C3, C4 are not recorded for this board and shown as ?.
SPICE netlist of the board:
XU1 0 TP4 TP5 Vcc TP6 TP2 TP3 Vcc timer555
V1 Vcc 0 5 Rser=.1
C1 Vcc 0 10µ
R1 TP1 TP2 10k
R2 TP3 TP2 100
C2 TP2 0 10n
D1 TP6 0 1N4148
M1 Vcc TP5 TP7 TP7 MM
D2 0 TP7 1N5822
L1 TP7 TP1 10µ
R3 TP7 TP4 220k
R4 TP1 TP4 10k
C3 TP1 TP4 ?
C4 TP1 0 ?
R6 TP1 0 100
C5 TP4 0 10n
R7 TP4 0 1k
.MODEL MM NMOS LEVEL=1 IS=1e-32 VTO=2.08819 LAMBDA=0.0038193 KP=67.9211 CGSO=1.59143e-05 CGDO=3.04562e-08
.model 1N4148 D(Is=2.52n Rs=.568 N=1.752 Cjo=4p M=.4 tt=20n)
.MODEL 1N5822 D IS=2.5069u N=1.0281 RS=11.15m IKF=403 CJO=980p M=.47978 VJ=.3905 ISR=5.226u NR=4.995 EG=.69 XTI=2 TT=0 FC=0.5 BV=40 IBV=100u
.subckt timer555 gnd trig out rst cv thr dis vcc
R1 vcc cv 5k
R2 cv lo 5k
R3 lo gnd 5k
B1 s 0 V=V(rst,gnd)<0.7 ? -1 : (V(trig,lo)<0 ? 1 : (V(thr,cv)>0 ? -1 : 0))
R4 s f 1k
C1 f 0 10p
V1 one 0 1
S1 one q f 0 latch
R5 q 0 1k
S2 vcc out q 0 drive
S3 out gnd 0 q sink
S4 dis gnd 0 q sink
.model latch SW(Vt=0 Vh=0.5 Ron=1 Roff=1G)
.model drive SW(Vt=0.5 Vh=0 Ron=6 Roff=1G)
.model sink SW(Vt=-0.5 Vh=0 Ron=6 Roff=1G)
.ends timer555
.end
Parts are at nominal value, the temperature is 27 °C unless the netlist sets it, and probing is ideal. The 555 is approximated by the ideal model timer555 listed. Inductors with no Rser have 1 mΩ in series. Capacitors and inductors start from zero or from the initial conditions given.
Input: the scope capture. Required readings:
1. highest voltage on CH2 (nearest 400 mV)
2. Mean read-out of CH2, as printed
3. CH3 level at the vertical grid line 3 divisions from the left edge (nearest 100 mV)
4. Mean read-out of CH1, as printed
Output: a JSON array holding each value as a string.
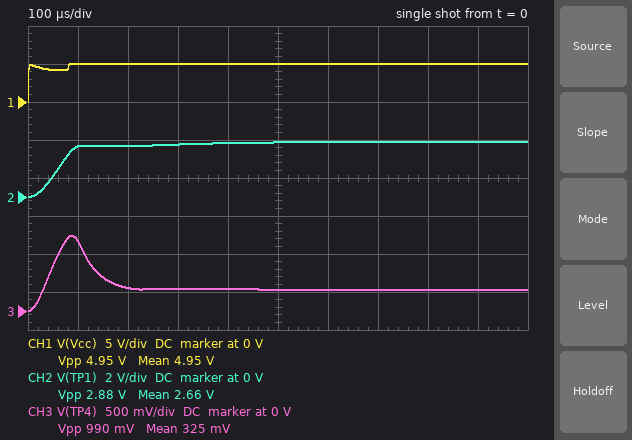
["2.8 V", "2.66 V", "300 mV", "4.95 V"]
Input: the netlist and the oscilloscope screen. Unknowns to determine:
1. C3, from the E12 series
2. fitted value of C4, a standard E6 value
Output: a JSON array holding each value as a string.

["33 nF", "220 µF"]
